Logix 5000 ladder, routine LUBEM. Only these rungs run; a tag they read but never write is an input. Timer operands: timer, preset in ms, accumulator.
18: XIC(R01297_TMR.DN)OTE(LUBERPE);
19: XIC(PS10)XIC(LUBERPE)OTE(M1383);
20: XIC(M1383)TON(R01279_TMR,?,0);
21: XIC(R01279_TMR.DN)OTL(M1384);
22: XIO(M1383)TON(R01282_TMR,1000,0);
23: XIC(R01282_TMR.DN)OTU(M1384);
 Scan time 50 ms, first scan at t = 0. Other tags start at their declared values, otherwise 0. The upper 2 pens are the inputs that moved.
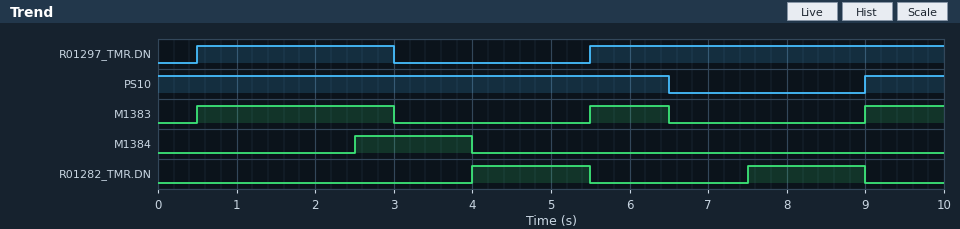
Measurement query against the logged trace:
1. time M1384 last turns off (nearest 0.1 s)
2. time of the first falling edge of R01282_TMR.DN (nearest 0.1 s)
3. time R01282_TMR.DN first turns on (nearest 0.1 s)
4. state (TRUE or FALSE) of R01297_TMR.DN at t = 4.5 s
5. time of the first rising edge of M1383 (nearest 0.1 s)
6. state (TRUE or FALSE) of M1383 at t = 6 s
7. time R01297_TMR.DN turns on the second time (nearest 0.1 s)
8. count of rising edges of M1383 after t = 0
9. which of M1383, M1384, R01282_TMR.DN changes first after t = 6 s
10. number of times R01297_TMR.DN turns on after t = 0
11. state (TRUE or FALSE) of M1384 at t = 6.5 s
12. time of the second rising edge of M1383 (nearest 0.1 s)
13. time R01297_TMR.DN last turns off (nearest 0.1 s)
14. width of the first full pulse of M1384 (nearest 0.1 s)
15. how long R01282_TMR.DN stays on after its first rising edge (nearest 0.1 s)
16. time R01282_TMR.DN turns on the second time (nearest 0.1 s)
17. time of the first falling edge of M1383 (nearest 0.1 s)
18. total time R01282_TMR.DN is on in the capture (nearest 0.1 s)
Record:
4.0 s
5.5 s
4.0 s
FALSE
0.5 s
TRUE
5.5 s
3
M1383
2
FALSE
5.5 s
3.0 s
1.5 s
1.5 s
7.5 s
3.0 s
3.0 s
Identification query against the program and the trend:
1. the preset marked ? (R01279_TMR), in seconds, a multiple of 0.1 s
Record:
2.0 s
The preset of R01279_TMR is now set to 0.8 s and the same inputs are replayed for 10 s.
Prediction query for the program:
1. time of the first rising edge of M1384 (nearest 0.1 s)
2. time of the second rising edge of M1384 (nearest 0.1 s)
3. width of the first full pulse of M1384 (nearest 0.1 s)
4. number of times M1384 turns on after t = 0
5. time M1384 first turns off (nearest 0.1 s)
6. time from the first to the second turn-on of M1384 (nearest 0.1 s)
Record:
1.3 s
6.3 s
2.7 s
3
4.0 s
5.0 s
